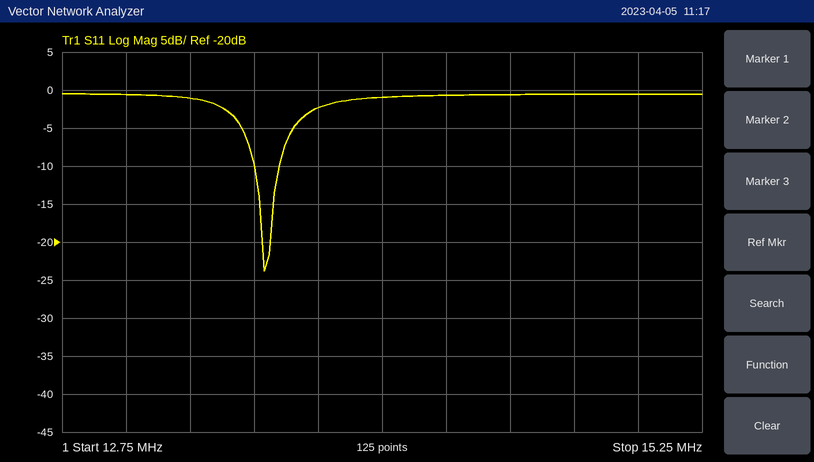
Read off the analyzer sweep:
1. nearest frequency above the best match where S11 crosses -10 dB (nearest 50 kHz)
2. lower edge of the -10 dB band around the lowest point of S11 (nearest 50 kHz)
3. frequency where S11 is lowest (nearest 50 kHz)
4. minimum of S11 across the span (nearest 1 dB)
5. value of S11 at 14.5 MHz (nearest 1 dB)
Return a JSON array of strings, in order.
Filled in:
["13.60 MHz", "13.50 MHz", "13.55 MHz", "-24 dB", "-1 dB"]
